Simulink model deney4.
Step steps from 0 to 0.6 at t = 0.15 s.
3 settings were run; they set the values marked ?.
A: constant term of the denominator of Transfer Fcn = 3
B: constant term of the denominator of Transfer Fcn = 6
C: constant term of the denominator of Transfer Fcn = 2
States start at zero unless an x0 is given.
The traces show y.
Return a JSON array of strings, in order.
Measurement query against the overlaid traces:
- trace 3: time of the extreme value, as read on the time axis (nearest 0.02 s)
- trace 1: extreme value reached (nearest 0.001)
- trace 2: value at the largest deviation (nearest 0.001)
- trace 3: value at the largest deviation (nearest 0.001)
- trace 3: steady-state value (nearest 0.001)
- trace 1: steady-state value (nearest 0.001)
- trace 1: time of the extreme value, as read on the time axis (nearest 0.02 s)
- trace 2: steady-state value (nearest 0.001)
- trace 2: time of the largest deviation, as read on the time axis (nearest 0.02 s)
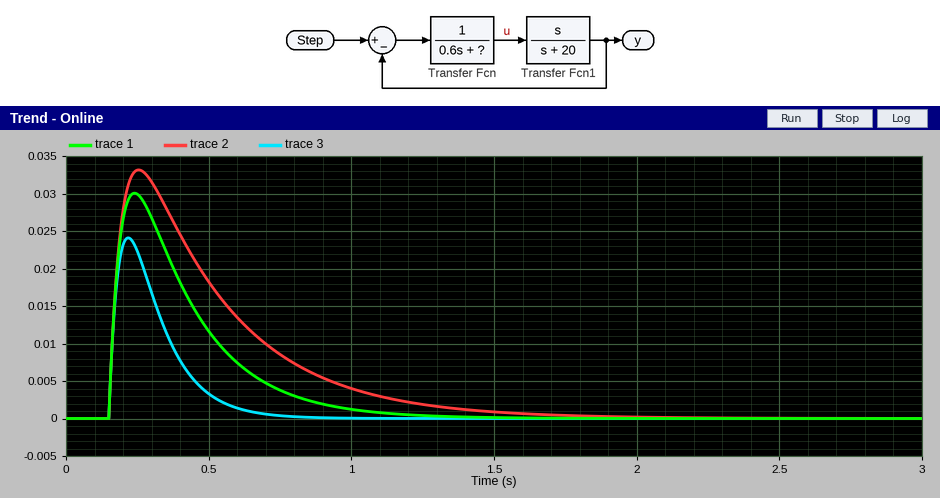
["0.22 s", "0.030", "0.033", "0.024", "0.000", "0.000", "0.24 s", "0.000", "0.26 s"]
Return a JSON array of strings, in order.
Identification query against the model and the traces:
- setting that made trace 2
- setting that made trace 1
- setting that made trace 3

["C", "A", "B"]
